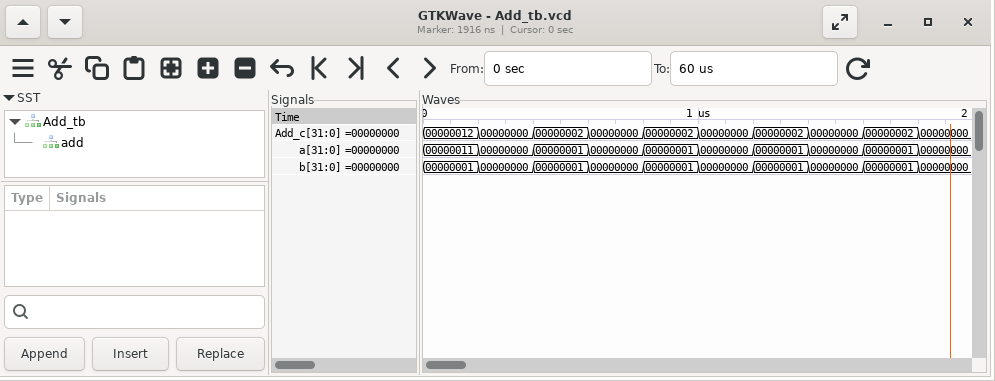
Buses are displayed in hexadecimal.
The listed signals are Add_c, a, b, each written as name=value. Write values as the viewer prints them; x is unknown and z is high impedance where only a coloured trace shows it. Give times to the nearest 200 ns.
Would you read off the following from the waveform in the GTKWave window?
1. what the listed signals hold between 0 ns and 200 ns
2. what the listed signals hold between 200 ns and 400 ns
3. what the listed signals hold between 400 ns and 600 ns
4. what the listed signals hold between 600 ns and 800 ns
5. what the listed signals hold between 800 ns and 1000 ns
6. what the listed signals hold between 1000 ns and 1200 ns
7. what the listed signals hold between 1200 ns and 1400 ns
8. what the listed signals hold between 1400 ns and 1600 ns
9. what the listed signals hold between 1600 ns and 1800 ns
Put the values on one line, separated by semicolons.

Add_c=00000012, a=00000011, b=00000001; Add_c=00000000, a=00000000, b=00000000; Add_c=00000002, a=00000001, b=00000001; Add_c=00000000, a=00000000, b=00000000; Add_c=00000002, a=00000001, b=00000001; Add_c=00000000, a=00000000, b=00000000; Add_c=00000002, a=00000001, b=00000001; Add_c=00000000, a=00000000, b=00000000; Add_c=00000002, a=00000001, b=00000001
